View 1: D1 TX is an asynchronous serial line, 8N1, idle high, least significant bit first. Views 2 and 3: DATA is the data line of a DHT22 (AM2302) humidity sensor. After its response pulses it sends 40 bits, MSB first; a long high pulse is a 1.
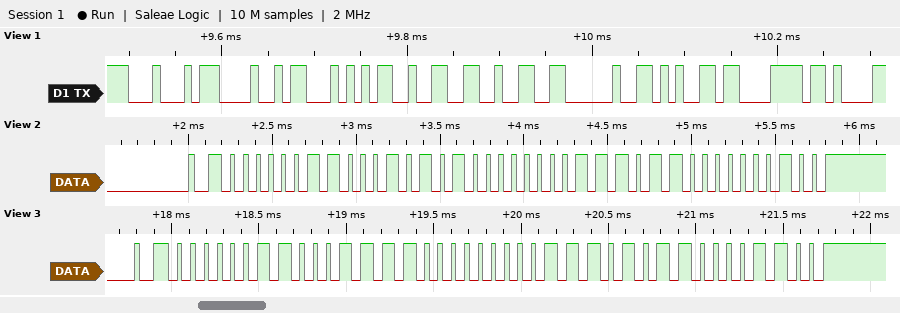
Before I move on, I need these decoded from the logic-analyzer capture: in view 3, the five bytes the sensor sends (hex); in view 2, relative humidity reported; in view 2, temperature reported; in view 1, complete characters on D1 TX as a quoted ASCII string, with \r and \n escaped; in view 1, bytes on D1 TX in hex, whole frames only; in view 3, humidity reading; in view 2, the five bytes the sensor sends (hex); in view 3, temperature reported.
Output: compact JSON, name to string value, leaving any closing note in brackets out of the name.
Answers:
{"in view 3, the five bytes the sensor sends": "03 1E 00 EB 0C", "in view 2, relative humidity reported": "78.9 %", "in view 2, temperature reported": "23.6 °C", "in view 1, complete characters on D1 TX as a quoted ASCII string, with \\r and \\n escaped": "\"DHT22 ex\"", "in view 1, bytes on D1 TX in hex, whole frames only": "0x44 0x48 0x54 0x32 0x32 0x20 0x65 0x78", "in view 3, humidity reading": "79.8 %", "in view 2, the five bytes the sensor sends": "03 15 00 EC 04", "in view 3, temperature reported": "23.5 °C"}
